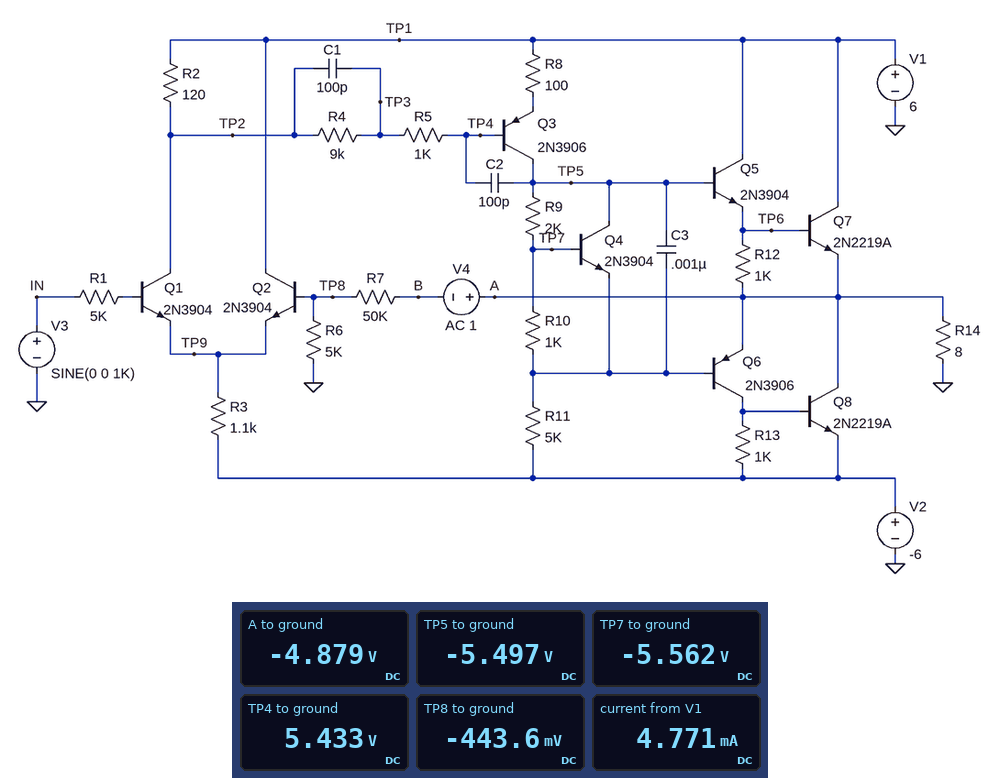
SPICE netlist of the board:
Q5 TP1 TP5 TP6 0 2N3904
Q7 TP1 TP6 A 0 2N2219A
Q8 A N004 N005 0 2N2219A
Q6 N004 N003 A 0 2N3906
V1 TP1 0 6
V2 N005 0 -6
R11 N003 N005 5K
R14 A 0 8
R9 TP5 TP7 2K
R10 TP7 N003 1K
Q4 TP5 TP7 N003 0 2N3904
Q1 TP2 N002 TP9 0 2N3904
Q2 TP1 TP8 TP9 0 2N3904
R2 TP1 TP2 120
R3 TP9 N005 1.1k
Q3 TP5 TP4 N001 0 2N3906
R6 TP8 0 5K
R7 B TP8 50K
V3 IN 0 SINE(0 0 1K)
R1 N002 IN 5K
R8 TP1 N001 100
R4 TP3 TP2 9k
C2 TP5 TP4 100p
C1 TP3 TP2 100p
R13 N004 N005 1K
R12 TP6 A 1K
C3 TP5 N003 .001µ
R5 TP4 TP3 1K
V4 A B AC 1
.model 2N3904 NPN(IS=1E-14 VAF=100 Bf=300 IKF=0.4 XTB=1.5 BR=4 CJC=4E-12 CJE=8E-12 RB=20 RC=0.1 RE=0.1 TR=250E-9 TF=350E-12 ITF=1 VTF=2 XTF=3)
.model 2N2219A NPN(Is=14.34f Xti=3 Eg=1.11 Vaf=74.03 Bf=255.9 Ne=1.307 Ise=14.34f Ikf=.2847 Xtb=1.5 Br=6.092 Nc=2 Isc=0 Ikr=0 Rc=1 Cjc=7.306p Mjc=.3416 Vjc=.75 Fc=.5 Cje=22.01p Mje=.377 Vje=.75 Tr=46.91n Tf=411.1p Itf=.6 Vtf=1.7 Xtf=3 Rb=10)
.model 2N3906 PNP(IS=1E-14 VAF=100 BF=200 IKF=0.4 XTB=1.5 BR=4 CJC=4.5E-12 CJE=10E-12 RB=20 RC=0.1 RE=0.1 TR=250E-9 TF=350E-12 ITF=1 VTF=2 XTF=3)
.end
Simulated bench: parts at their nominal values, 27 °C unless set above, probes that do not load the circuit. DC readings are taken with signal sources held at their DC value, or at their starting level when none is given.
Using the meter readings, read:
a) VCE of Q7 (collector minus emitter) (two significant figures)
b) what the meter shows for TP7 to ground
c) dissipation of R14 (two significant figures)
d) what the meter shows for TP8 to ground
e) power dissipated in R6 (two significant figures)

11 V
-5.562 V
3.0 W
-443.6 mV
39 µW
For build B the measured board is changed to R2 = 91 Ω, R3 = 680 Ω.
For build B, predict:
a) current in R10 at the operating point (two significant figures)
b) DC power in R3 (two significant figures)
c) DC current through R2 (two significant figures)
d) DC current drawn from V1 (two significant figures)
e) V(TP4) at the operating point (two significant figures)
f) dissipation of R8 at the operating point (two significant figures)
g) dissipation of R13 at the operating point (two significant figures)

400 µA
39 mW
7.6 mA
8.0 mA
5.3 V
16 µW
740 µW
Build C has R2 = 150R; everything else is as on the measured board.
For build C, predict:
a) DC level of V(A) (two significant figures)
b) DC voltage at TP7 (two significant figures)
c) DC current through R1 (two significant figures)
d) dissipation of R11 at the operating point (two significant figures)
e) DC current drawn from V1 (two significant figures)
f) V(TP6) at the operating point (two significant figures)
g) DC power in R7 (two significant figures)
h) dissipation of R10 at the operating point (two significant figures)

-2.7 V
-2.9 V
15 µA
1.4 mW
5.4 mA
-2.5 V
120 µW
250 µW
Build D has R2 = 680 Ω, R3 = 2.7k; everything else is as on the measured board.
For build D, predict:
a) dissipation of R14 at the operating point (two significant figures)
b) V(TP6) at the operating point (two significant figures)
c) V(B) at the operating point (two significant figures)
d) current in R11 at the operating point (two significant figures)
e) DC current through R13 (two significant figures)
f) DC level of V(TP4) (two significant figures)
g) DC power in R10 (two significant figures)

5.7 mW
390 mV
-210 mV
1.0 mA
730 µA
5.2 V
400 µW
